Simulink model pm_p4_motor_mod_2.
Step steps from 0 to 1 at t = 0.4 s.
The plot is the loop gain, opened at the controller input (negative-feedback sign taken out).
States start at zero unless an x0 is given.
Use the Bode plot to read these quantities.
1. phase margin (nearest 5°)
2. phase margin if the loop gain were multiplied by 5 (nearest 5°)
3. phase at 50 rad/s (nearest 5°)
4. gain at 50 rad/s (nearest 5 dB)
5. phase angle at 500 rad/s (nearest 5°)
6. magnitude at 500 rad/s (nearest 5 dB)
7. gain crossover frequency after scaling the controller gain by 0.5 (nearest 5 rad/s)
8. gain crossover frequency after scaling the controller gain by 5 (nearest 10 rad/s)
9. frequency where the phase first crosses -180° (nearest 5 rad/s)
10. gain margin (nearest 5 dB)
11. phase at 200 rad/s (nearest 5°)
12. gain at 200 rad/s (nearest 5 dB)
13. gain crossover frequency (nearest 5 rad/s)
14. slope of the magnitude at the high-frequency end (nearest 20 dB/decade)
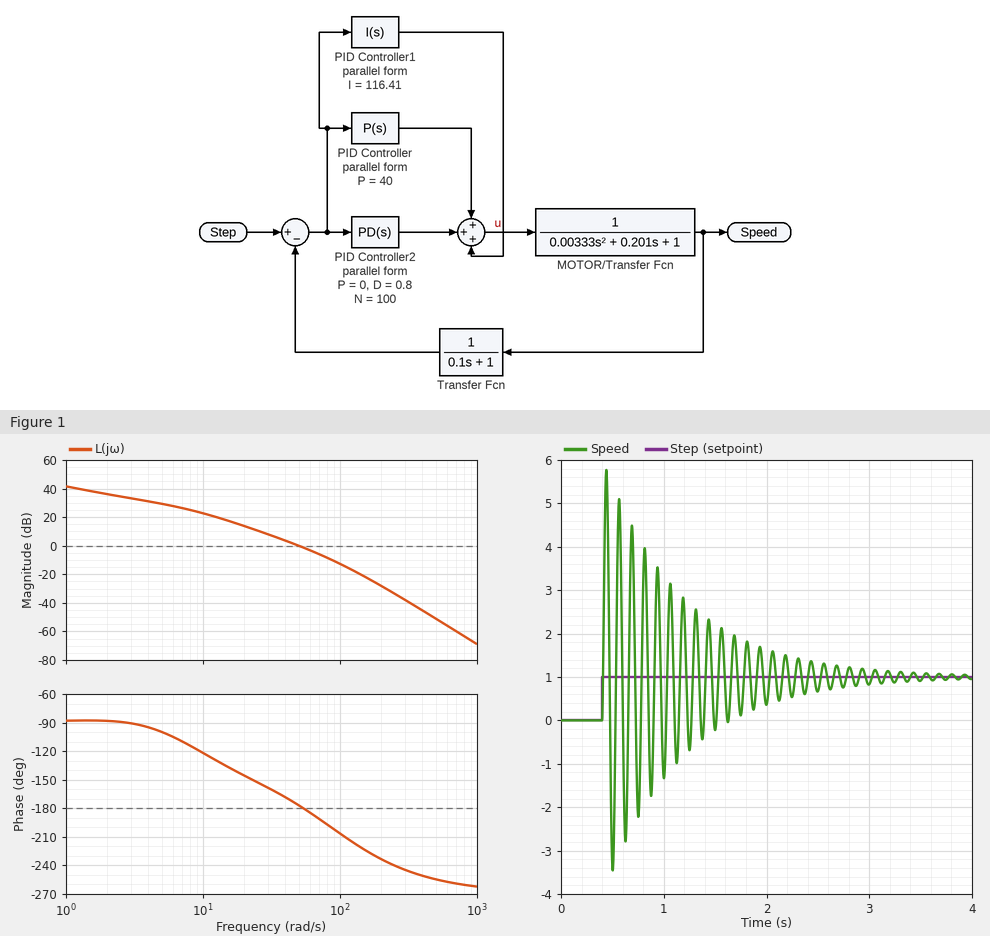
5°
-30°
-175°
0 dB
-255°
-50 dB
35 rad/s
110 rad/s
55 rad/s
0 dB
-235°
-30 dB
50 rad/s
-60 dB/decade
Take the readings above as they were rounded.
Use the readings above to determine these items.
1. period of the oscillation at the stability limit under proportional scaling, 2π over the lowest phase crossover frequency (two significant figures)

0.11 s
